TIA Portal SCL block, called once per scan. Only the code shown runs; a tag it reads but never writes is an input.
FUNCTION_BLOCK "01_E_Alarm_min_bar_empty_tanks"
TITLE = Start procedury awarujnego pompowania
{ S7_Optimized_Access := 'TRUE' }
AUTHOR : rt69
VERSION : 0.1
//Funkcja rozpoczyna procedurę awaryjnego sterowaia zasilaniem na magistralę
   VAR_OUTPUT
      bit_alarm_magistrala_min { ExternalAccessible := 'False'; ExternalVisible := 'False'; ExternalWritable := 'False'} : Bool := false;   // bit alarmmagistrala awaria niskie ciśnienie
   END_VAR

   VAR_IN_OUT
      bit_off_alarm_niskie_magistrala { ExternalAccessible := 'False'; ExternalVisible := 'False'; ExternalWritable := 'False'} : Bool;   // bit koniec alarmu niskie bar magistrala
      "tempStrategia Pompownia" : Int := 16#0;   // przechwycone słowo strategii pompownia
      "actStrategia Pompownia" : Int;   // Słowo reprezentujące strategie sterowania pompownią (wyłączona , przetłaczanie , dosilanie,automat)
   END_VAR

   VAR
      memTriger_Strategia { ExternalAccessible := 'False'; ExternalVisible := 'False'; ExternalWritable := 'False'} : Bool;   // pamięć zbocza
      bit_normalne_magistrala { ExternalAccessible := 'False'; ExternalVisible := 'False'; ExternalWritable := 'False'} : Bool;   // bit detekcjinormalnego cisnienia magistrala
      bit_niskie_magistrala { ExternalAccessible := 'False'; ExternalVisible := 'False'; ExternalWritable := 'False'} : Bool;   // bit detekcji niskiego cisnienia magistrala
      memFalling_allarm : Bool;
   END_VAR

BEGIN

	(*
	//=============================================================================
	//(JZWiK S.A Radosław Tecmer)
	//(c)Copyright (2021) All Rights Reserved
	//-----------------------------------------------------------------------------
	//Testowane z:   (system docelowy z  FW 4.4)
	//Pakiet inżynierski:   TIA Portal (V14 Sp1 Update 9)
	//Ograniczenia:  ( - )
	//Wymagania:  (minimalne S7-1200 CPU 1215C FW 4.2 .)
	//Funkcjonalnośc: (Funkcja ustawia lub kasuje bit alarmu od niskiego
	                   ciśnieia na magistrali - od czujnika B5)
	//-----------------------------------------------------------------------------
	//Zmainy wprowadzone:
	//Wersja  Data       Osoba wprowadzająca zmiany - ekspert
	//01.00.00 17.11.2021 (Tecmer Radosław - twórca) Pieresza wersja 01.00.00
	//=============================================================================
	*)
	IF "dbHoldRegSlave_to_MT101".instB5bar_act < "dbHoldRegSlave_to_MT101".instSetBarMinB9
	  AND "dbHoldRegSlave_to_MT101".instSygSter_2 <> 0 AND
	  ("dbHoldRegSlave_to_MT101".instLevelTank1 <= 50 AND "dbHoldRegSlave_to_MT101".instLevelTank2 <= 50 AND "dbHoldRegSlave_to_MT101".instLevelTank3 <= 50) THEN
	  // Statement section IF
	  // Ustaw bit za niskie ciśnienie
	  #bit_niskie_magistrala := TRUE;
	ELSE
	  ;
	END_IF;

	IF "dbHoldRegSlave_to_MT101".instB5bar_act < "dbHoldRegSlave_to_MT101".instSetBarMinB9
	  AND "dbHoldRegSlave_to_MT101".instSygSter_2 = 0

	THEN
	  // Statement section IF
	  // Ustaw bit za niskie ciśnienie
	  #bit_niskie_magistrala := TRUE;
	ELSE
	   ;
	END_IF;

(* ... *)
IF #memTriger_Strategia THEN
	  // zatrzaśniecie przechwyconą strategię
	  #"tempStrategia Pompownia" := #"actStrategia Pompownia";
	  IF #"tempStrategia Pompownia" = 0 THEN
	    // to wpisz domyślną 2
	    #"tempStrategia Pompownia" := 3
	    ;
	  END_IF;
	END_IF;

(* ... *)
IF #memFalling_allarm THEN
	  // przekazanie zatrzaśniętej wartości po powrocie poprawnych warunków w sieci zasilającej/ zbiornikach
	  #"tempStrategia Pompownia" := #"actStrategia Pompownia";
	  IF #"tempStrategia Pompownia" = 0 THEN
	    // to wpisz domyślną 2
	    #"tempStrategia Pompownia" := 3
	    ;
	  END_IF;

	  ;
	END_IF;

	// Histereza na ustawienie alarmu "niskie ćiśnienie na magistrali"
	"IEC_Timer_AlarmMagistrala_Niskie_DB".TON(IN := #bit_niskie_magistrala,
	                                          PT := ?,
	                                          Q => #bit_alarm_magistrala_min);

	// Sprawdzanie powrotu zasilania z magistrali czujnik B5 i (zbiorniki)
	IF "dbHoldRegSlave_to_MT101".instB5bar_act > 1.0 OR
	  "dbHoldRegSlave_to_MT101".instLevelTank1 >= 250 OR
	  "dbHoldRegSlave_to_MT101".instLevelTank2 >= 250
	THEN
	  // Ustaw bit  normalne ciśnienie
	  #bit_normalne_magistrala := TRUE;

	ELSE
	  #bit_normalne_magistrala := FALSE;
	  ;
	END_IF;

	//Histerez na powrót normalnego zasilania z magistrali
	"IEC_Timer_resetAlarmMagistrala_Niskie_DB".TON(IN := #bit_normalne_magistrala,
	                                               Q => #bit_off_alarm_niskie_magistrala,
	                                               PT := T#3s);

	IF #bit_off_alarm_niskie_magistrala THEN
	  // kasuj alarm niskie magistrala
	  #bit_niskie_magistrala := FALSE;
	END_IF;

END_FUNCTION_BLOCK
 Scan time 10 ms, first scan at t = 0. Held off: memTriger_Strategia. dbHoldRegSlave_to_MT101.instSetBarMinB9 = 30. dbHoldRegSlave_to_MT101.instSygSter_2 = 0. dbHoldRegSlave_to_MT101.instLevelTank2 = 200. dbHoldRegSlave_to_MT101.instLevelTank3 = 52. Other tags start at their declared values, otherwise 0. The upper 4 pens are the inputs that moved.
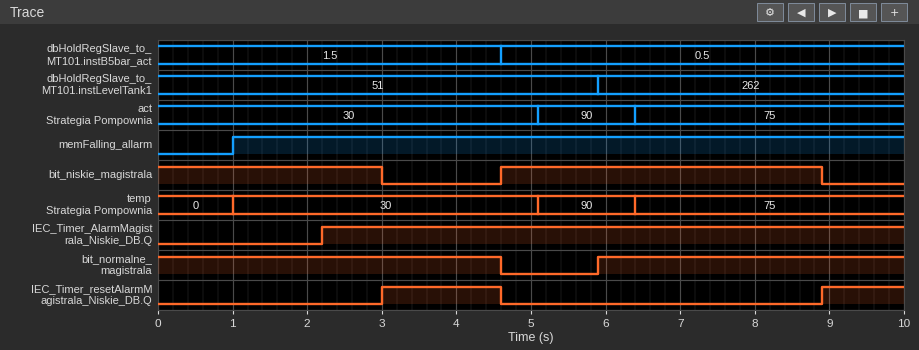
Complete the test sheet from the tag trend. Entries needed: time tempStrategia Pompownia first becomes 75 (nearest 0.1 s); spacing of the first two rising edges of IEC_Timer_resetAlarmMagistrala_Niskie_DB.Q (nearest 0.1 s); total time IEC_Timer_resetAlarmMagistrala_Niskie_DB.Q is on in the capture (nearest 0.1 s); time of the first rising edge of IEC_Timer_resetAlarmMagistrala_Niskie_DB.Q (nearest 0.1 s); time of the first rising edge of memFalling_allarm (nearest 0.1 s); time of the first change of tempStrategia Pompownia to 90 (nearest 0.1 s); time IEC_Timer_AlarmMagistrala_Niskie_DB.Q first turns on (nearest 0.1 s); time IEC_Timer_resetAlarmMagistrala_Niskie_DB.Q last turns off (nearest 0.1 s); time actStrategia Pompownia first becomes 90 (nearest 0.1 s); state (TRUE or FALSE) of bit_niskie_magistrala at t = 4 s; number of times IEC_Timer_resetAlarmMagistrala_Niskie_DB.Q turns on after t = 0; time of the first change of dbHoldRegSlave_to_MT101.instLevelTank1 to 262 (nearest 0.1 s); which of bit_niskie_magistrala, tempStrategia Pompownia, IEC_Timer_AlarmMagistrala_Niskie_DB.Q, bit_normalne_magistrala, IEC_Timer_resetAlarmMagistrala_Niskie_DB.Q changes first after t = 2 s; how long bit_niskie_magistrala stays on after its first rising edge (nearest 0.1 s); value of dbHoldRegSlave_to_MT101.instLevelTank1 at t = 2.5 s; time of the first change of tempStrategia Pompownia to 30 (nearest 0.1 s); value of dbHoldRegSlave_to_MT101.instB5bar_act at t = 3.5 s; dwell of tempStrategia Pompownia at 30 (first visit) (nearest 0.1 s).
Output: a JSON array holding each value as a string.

["6.4 s", "5.9 s", "2.7 s", "3.0 s", "1.0 s", "5.1 s", "2.2 s", "4.6 s", "5.1 s", "FALSE", "2", "5.9 s", "IEC_Timer_AlarmMagistrala_Niskie_DB.Q", "4.3 s", "51", "1.0 s", "1.5", "4.1 s"]
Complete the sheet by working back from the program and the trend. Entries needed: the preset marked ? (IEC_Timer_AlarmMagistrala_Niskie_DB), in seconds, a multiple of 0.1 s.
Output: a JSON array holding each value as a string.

["2.2 s"]
